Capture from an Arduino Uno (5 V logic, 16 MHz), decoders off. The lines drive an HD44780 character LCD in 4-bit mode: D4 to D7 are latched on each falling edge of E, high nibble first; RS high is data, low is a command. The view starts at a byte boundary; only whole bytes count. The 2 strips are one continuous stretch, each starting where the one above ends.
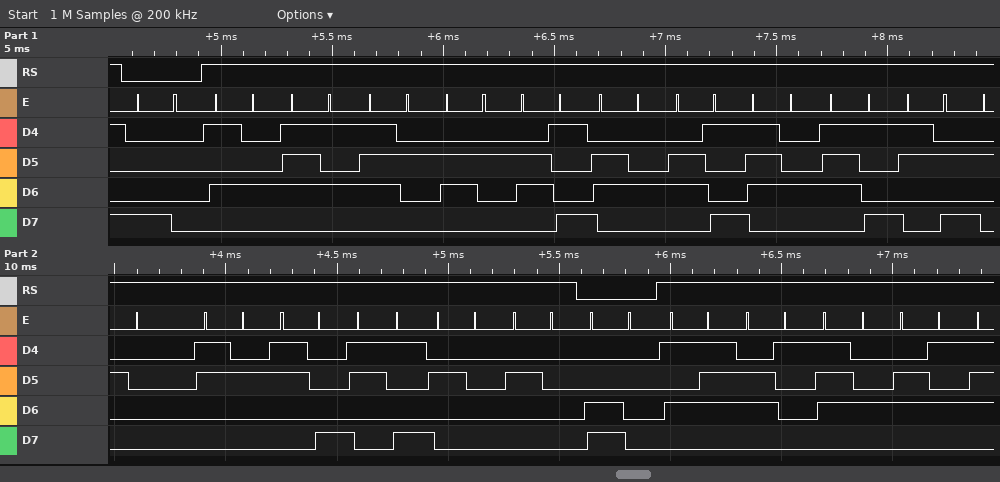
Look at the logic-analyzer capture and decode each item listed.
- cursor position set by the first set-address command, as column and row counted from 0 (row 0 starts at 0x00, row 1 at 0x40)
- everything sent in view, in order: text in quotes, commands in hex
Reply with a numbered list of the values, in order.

1. column 0, row 0
2. 0x80 "Turbidity: 289  " 0xC0 "Wate"
